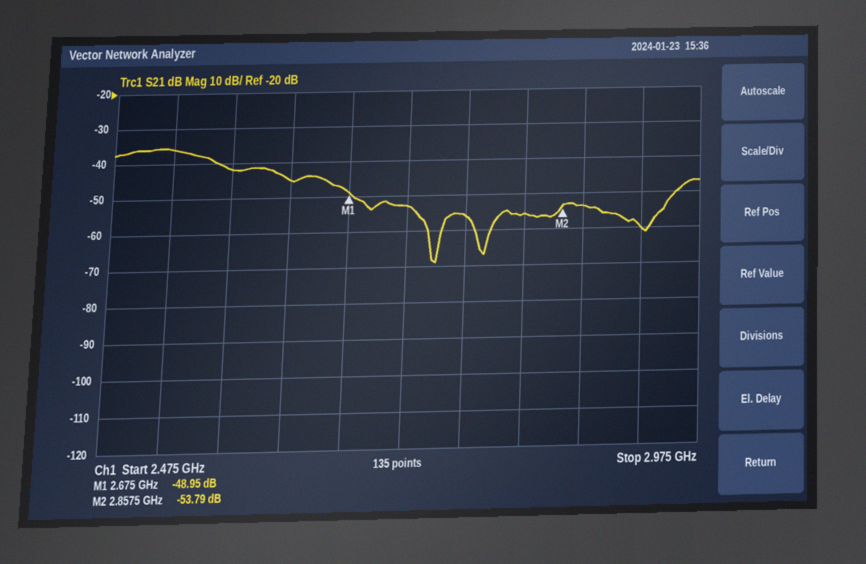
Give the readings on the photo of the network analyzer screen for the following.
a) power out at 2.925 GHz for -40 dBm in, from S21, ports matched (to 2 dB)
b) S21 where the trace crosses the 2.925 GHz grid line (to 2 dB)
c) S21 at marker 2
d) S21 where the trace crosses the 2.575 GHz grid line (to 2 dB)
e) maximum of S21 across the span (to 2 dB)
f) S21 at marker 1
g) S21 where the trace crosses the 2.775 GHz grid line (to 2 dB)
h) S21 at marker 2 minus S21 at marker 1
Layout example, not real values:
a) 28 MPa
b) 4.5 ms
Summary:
a) -100 dBm
b) -60 dB
c) -53.79 dB
d) -42 dB
e) -36 dB
f) -48.95 dB
g) -56 dB
h) -4.84 dB
